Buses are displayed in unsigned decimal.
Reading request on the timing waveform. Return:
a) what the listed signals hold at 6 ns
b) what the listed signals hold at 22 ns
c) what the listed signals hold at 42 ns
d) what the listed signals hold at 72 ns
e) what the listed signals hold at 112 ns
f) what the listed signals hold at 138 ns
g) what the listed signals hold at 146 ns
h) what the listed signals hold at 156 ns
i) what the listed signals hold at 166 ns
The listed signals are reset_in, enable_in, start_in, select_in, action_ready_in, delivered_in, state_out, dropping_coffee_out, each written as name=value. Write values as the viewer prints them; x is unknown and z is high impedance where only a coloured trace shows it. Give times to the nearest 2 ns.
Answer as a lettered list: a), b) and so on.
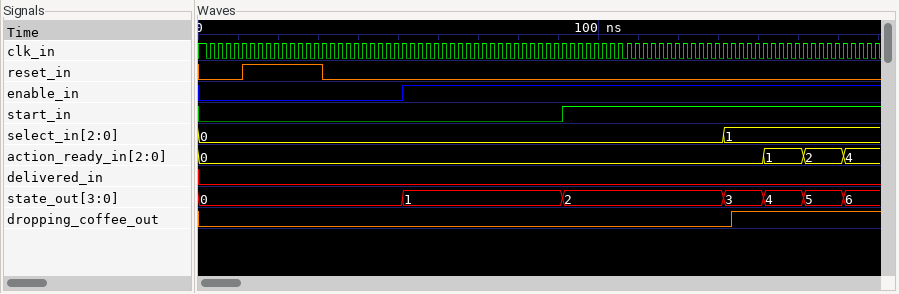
a) reset_in=0, enable_in=0, start_in=0, select_in=0, action_ready_in=0, delivered_in=0, state_out=0, dropping_coffee_out=0
b) reset_in=1, enable_in=0, start_in=0, select_in=0, action_ready_in=0, delivered_in=0, state_out=0, dropping_coffee_out=0
c) reset_in=0, enable_in=0, start_in=0, select_in=0, action_ready_in=0, delivered_in=0, state_out=0, dropping_coffee_out=0
d) reset_in=0, enable_in=1, start_in=0, select_in=0, action_ready_in=0, delivered_in=0, state_out=1, dropping_coffee_out=0
e) reset_in=0, enable_in=1, start_in=1, select_in=0, action_ready_in=0, delivered_in=0, state_out=2, dropping_coffee_out=0
f) reset_in=0, enable_in=1, start_in=1, select_in=1, action_ready_in=0, delivered_in=0, state_out=3, dropping_coffee_out=1
g) reset_in=0, enable_in=1, start_in=1, select_in=1, action_ready_in=1, delivered_in=0, state_out=4, dropping_coffee_out=1
h) reset_in=0, enable_in=1, start_in=1, select_in=1, action_ready_in=2, delivered_in=0, state_out=5, dropping_coffee_out=1
i) reset_in=0, enable_in=1, start_in=1, select_in=1, action_ready_in=4, delivered_in=0, state_out=6, dropping_coffee_out=1
